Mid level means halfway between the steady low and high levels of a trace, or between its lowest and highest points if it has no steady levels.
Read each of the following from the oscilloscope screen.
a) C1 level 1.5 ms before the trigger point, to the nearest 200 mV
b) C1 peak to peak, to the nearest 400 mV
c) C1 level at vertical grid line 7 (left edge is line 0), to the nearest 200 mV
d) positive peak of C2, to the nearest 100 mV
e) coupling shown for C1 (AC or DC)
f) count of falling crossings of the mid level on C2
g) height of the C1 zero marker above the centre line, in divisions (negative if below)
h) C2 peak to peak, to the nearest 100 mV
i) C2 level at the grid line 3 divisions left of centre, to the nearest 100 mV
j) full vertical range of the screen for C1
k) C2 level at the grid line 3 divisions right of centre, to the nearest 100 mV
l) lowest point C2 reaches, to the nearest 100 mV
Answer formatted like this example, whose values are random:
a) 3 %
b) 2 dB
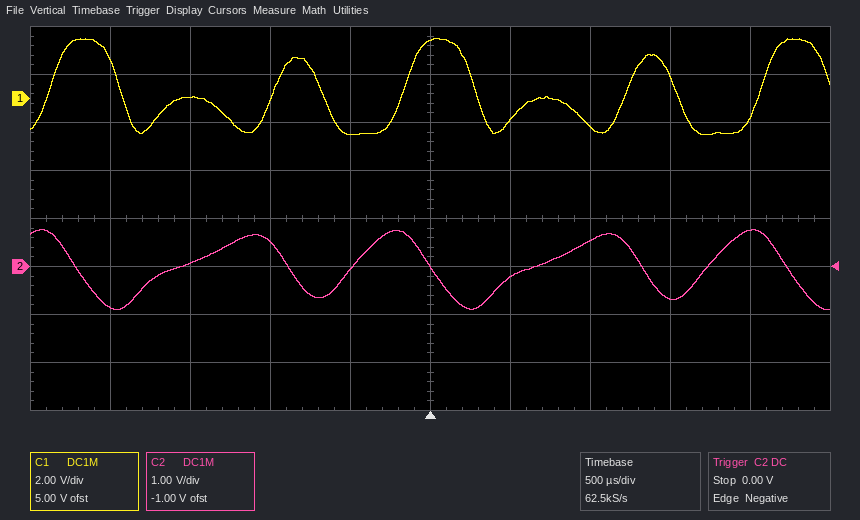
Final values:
a) 0.0 V
b) 4.0 V
c) -1.2 V
d) 800 mV
e) DC
f) 5
g) +2.5 div
h) 1.7 V
i) 100 mV
j) 16 V
k) -700 mV
l) -900 mV
